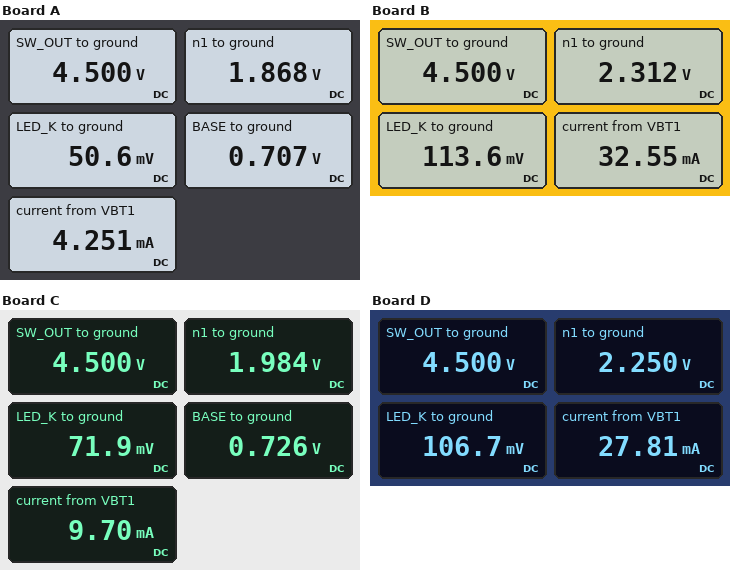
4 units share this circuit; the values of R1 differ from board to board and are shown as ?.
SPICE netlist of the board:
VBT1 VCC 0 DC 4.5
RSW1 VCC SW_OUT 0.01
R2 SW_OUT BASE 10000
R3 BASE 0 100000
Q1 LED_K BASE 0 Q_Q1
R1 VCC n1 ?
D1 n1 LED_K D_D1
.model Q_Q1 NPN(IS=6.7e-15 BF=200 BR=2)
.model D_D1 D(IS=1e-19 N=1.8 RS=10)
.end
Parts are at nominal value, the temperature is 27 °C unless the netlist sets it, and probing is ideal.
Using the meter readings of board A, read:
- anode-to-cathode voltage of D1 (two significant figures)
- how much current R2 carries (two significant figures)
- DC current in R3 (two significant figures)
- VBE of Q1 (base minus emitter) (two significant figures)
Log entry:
1.8 V
380 µA
7.1 µA
710 mV
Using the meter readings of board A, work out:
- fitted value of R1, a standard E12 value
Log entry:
680 Ω
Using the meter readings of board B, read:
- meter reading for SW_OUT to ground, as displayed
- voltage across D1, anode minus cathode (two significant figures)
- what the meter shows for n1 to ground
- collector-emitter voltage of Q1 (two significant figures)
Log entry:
4.500 V
2.2 V
2.312 V
110 mV
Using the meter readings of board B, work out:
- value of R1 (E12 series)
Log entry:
68 Ω
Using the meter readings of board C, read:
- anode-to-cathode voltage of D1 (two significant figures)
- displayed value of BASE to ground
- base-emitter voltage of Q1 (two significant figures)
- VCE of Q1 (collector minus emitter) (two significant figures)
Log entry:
1.9 V
0.726 V
730 mV
72 mV
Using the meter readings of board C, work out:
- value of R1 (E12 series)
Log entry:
270 Ω
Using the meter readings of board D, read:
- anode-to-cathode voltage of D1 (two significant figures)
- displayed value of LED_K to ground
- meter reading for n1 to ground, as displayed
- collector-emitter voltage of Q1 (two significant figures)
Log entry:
2.1 V
106.7 mV
2.250 V
110 mV
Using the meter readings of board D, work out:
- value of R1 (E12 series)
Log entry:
82 Ω
